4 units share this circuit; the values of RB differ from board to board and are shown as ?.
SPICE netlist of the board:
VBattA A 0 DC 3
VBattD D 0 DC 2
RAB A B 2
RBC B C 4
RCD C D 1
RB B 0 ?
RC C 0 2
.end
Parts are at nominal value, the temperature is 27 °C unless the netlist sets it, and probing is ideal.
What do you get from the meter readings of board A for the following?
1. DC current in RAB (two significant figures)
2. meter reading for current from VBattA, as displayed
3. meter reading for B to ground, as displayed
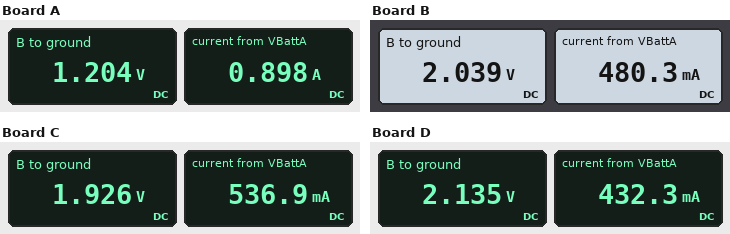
900 mA
0.898 A
1.204 V
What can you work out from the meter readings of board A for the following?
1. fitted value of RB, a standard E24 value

1.3 Ω
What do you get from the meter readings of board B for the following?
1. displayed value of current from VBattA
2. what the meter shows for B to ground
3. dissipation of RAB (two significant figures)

480.3 mA
2.039 V
460 mW
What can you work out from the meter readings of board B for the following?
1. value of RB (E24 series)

6.2 Ω
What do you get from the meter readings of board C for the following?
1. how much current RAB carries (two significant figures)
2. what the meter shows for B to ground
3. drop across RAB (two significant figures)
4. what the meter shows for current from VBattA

540 mA
1.926 V
1.1 V
536.9 mA
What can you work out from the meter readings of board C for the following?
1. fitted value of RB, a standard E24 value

4.7 Ω
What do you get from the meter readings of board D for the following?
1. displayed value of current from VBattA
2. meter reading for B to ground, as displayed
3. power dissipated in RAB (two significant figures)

432.3 mA
2.135 V
370 mW
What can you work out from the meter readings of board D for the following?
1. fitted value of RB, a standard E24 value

8.2 Ω
